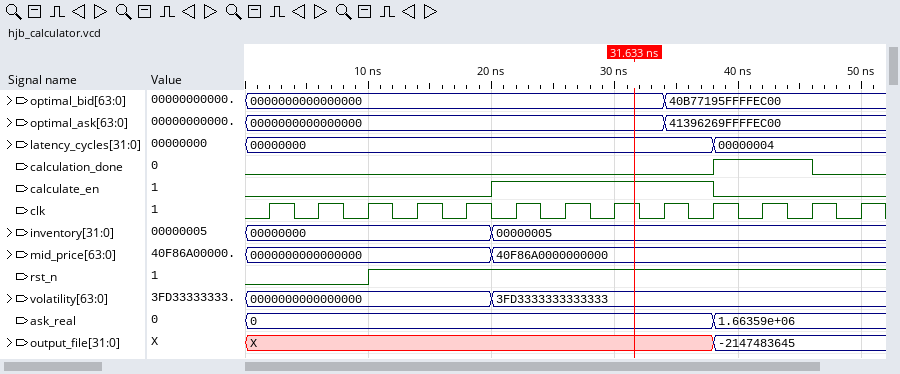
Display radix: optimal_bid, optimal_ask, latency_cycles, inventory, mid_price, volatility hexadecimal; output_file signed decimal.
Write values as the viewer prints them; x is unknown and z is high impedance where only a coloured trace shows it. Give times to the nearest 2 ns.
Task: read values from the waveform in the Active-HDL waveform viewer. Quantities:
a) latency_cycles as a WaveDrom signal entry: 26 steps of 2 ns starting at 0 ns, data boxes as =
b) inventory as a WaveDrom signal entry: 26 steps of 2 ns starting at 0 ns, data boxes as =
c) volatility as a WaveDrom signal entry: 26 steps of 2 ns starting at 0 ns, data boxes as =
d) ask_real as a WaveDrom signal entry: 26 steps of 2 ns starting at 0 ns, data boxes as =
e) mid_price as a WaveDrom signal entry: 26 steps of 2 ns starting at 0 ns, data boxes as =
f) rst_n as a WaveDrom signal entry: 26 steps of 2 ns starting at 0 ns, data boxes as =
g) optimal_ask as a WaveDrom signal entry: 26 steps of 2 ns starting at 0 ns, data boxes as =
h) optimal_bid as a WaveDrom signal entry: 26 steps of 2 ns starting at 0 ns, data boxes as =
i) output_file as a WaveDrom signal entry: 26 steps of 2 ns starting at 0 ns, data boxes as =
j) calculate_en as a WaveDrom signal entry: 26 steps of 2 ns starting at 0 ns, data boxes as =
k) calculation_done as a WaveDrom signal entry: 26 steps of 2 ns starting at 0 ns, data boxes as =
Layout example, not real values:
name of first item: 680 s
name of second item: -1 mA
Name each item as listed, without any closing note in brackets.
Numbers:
latency_cycles as a WaveDrom signal entry: 26 steps of 2 ns starting at 0 ns, data boxes as =: {name: 'latency_cycles', wave: '=..................=......', data: '00000000 00000004'}
inventory as a WaveDrom signal entry: 26 steps of 2 ns starting at 0 ns, data boxes as =: {name: 'inventory', wave: '=.........=...............', data: '00000000 00000005'}
volatility as a WaveDrom signal entry: 26 steps of 2 ns starting at 0 ns, data boxes as =: {name: 'volatility', wave: '=.........=...............', data: '0000000000000000 3FD3333333333333'}
ask_real as a WaveDrom signal entry: 26 steps of 2 ns starting at 0 ns, data boxes as =: {name: 'ask_real', wave: '=..................=......', data: '0 1.66359e+06'}
mid_price as a WaveDrom signal entry: 26 steps of 2 ns starting at 0 ns, data boxes as =: {name: 'mid_price', wave: '=.........=...............', data: '0000000000000000 40F86A0000000000'}
rst_n as a WaveDrom signal entry: 26 steps of 2 ns starting at 0 ns, data boxes as =: {name: 'rst_n', wave: '0....1....................'}
optimal_ask as a WaveDrom signal entry: 26 steps of 2 ns starting at 0 ns, data boxes as =: {name: 'optimal_ask', wave: '=................=........', data: '0000000000000000 41396269FFFFEC00'}
optimal_bid as a WaveDrom signal entry: 26 steps of 2 ns starting at 0 ns, data boxes as =: {name: 'optimal_bid', wave: '=................=........', data: '0000000000000000 40B77195FFFFEC00'}
output_file as a WaveDrom signal entry: 26 steps of 2 ns starting at 0 ns, data boxes as =: {name: 'output_file', wave: 'x..................=......', data: '-2147483645'}
calculate_en as a WaveDrom signal entry: 26 steps of 2 ns starting at 0 ns, data boxes as =: {name: 'calculate_en', wave: '0.........1........0......'}
calculation_done as a WaveDrom signal entry: 26 steps of 2 ns starting at 0 ns, data boxes as =: {name: 'calculation_done', wave: '0..................1...0..'}
